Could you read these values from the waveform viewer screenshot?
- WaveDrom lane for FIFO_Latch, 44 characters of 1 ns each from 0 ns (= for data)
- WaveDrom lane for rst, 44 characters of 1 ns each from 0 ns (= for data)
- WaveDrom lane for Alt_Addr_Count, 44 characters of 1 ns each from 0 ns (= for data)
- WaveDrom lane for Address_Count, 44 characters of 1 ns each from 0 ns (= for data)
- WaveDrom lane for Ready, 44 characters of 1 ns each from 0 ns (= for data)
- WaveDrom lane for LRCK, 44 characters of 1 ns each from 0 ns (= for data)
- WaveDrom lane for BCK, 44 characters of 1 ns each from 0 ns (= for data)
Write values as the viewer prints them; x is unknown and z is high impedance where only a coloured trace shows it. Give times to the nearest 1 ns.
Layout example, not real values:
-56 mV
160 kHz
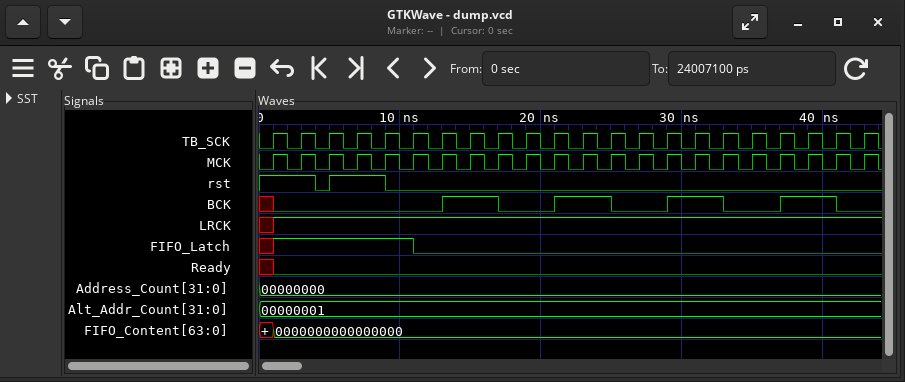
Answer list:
{name: 'FIFO_Latch', wave: 'x1.........0................................'}
{name: 'rst', wave: '1...01...0..................................'}
{name: 'Alt_Addr_Count', wave: '=...........................................', data: '00000001'}
{name: 'Address_Count', wave: '=...........................................', data: '00000000'}
{name: 'Ready', wave: 'x0..........................................'}
{name: 'LRCK', wave: 'x1..........................................'}
{name: 'BCK', wave: 'x0...........1...0...1...0...1...0...1...0..'}
